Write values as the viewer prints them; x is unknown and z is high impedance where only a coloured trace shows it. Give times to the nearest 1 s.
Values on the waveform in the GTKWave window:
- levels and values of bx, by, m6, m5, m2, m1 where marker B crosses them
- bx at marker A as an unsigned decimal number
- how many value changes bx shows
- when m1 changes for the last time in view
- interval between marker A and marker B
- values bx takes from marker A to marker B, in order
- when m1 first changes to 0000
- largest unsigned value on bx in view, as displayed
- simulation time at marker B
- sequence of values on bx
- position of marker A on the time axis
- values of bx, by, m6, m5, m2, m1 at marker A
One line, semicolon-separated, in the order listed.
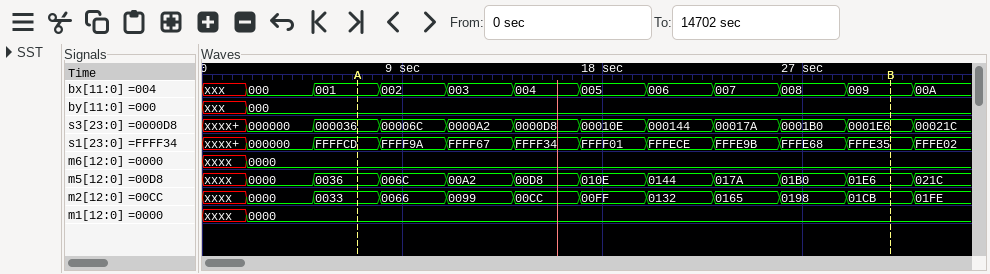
bx=009, by=000, m6=0000, m5=01E6, m2=01CB, m1=0000; 1; 11; 2 s; 24 s; 001, 002, 003, 004, 005, 006, 007, 008, 009; 2 s; 00A; 31 s; xxx, 000, 001, 002, 003, 004, 005, 006, 007, 008, 009, 00A; 7 s; bx=001, by=000, m6=0000, m5=0036, m2=0033, m1=0000
